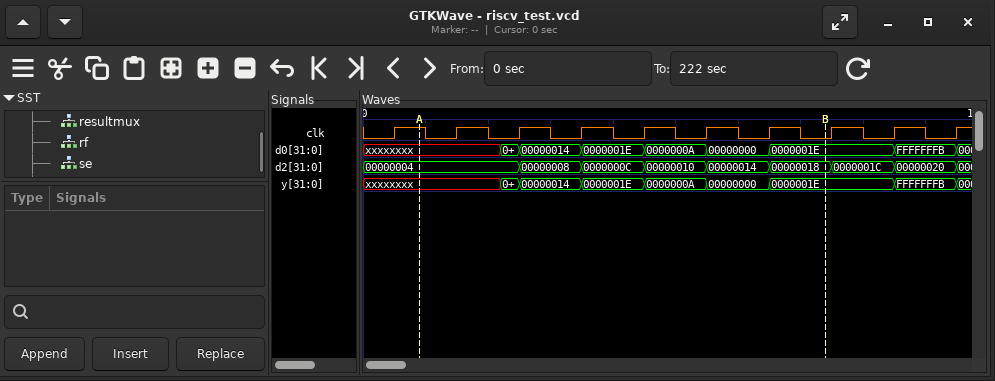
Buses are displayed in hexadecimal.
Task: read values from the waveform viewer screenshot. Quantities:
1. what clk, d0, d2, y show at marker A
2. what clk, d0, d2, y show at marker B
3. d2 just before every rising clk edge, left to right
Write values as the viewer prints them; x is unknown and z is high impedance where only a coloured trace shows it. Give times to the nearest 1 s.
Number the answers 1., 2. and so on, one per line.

1. clk=1, d0=xxxxxxxx, d2=00000004, y=xxxxxxxx
2. clk=0, d0=0000001E, d2=00000018, y=0000001E
3. 00000004, 00000004, 00000004, 00000008, 0000000C, 00000010, 00000014, 00000018, 0000001C, 00000020
